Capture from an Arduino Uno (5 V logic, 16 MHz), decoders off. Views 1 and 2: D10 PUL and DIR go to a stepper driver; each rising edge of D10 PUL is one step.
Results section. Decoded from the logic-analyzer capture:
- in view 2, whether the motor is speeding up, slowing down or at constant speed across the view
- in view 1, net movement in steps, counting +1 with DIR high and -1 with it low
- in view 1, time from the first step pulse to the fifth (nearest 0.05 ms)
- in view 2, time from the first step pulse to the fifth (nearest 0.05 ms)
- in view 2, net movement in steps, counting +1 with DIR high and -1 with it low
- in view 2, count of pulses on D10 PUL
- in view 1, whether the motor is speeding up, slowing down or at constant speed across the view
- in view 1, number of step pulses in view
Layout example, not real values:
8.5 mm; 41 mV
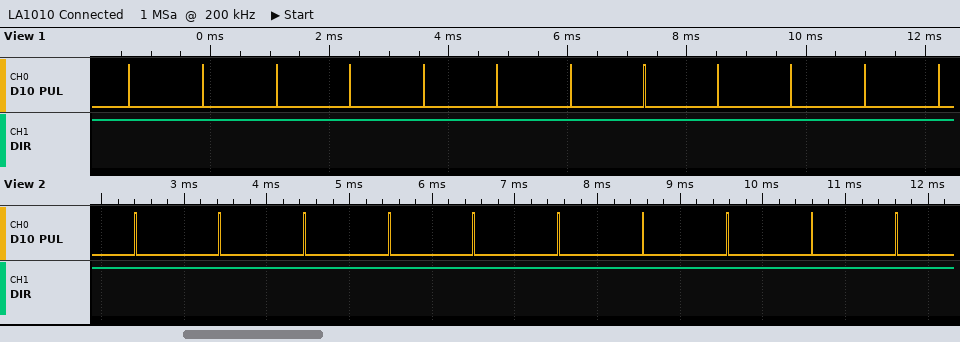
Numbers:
constant speed; +12; 4.95 ms; 4.10 ms; +10; 10; constant speed; 12
